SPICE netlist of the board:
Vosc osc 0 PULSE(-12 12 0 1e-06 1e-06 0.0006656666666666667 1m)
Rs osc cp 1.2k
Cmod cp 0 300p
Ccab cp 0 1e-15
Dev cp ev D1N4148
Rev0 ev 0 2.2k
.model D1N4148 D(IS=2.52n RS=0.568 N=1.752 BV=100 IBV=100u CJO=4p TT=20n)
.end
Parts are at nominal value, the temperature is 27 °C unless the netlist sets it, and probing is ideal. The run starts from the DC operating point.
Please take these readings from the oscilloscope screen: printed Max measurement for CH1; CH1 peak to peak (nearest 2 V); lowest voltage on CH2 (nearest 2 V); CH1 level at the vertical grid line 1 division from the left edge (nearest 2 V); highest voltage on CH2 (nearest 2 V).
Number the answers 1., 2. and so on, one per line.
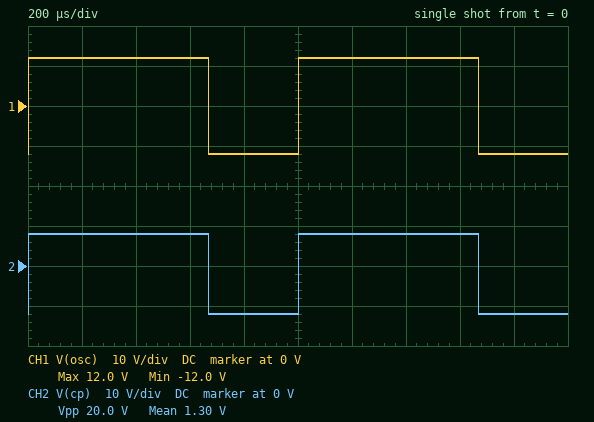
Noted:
1. 12.0 V
2. 24 V
3. -12 V
4. 12 V
5. 8 V
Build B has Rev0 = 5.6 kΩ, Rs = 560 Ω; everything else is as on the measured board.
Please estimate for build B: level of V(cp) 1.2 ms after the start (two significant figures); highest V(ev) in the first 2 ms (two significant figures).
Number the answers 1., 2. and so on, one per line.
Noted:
1. 11 V
2. 10 V
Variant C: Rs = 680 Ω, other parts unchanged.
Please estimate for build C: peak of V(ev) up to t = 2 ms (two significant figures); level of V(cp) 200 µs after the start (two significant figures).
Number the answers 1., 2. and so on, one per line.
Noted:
1. 8.7 V
2. 9.3 V
